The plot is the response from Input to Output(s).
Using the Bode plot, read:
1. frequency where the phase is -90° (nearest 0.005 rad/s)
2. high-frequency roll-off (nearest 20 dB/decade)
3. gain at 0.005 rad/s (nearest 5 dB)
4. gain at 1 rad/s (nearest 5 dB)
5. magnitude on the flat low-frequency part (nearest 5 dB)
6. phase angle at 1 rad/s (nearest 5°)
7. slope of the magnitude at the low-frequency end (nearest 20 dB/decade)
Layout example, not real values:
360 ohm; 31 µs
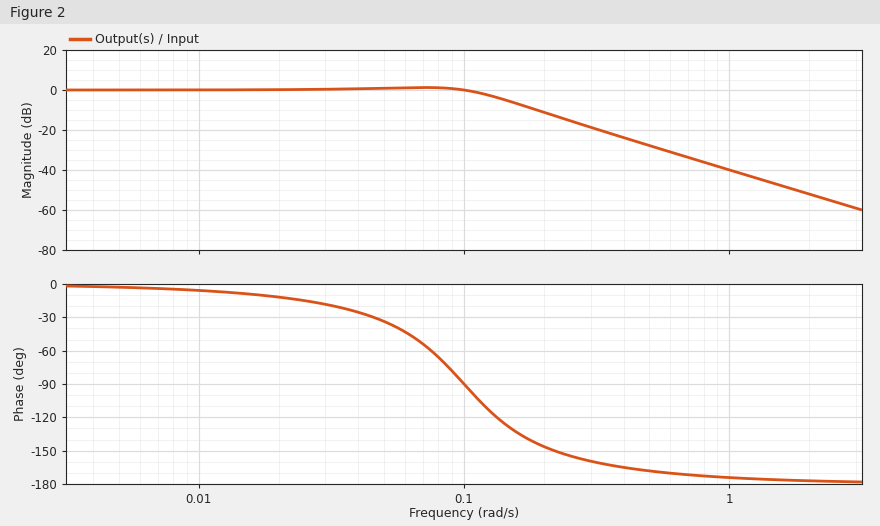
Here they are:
0.100 rad/s; -40 dB/decade; 0 dB; -40 dB; 0 dB; -175°; 0 dB/decade
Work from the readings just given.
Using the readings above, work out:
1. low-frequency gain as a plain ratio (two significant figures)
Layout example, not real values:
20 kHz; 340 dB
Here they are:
1.0
